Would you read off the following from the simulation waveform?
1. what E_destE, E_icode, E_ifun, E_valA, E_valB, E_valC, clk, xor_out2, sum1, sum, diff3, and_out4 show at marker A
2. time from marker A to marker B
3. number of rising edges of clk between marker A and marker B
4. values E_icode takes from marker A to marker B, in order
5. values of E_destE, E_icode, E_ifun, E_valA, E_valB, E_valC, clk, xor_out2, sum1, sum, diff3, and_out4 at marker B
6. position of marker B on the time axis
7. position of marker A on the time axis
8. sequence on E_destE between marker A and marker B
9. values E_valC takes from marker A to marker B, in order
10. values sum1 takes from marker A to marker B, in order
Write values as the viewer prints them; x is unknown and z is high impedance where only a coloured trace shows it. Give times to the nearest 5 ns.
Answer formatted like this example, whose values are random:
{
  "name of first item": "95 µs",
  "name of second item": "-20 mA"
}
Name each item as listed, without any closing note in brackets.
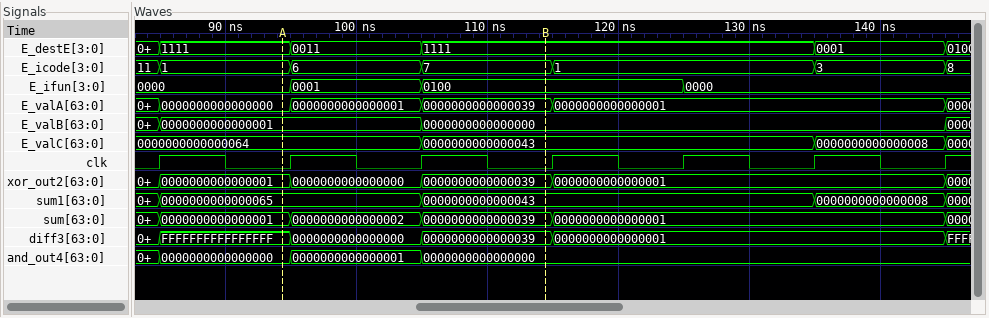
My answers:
{
  "what E_destE, E_icode, E_ifun, E_valA, E_valB, E_valC, clk, xor_out2, sum1, sum, diff3, and_out4 show at marker A": "E_destE=1111, E_icode=1, E_ifun=0000, E_valA=0000000000000000, E_valB=0000000000000001, E_valC=0000000000000064, clk=0, xor_out2=0000000000000001, sum1=0000000000000065, sum=0000000000000001, diff3=FFFFFFFFFFFFFFFF, and_out4=0000000000000000",
  "time from marker A to marker B": "20 ns",
  "number of rising edges of clk between marker A and marker B": "2",
  "values E_icode takes from marker A to marker B, in order": "1, 6, 7",
  "values of E_destE, E_icode, E_ifun, E_valA, E_valB, E_valC, clk, xor_out2, sum1, sum, diff3, and_out4 at marker B": "E_destE=1111, E_icode=7, E_ifun=0100, E_valA=0000000000000039, E_valB=0000000000000000, E_valC=0000000000000043, clk=0, xor_out2=0000000000000039, sum1=0000000000000043, sum=0000000000000039, diff3=0000000000000039, and_out4=0000000000000000",
  "position of marker B on the time axis": "115 ns",
  "position of marker A on the time axis": "95 ns",
  "sequence on E_destE between marker A and marker B": "1111, 0011, 1111",
  "values E_valC takes from marker A to marker B, in order": "0000000000000064, 0000000000000043",
  "values sum1 takes from marker A to marker B, in order": "0000000000000065, 0000000000000043"
}
